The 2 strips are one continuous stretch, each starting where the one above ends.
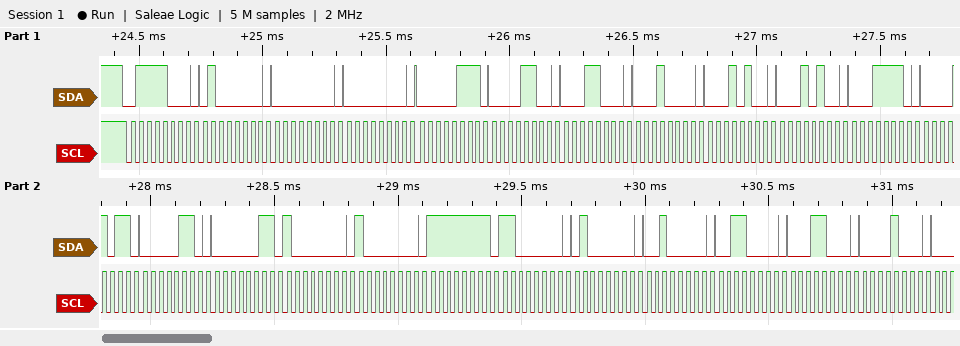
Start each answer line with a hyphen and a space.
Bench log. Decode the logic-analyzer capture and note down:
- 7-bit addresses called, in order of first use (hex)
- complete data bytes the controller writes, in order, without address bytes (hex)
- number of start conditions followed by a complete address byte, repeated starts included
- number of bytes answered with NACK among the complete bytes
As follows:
- 0x3C
- 40 00 00 07 0C 18 10 14 14 1E 0B 06 03 80 80 FF C0 40 20 30 18 08
- 1
- 0
